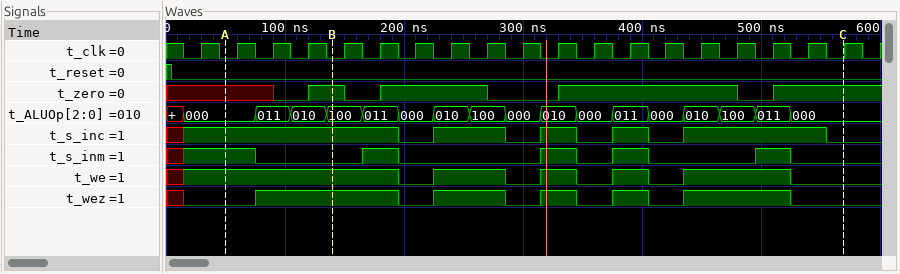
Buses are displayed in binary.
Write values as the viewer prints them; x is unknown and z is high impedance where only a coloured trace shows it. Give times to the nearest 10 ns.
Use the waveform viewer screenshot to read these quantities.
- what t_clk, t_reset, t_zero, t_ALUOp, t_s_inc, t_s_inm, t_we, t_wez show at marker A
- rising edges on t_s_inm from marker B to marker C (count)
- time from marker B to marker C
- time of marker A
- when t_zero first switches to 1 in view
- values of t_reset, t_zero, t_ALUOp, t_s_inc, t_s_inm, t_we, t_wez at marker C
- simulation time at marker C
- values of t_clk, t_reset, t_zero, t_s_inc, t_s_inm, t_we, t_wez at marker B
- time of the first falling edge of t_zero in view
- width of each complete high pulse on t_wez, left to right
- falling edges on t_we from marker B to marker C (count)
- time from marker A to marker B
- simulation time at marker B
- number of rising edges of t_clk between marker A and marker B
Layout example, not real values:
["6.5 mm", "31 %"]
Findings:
["t_clk=0, t_reset=0, t_zero=x, t_ALUOp=000, t_s_inc=1, t_s_inm=1, t_we=1, t_wez=0", "4", "430 ns", "50 ns", "120 ns", "t_reset=0, t_zero=1, t_ALUOp=000, t_s_inc=0, t_s_inm=0, t_we=0, t_wez=0", "570 ns", "t_clk=0, t_reset=0, t_zero=1, t_s_inc=1, t_s_inm=0, t_we=1, t_wez=1", "150 ns", "120 ns, 60 ns, 30 ns, 30 ns, 90 ns", "5", "90 ns", "140 ns", "3"]
